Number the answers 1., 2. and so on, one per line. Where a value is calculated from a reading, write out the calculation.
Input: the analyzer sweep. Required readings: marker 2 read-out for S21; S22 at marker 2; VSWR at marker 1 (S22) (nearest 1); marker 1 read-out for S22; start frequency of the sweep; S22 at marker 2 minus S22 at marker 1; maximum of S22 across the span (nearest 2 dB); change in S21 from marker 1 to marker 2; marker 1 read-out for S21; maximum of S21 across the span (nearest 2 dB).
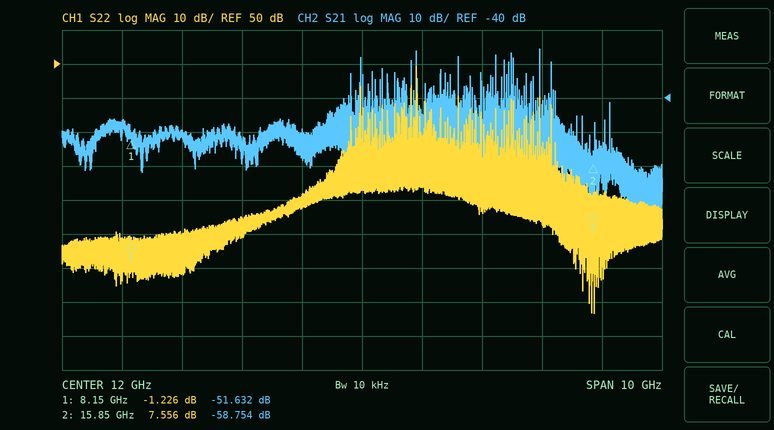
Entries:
1. -58.754 dB
2. 7.556 dB
3. (1 + 0.8684)/(1 − 0.8684) ≈ 14
4. -1.226 dB
5. 7 GHz
6. 7.556 − (-1.226) = 8.782 dB
7. 50 dB
8. -58.754 − (-51.632) = -7.122 dB
9. -51.632 dB
10. -26 dB
